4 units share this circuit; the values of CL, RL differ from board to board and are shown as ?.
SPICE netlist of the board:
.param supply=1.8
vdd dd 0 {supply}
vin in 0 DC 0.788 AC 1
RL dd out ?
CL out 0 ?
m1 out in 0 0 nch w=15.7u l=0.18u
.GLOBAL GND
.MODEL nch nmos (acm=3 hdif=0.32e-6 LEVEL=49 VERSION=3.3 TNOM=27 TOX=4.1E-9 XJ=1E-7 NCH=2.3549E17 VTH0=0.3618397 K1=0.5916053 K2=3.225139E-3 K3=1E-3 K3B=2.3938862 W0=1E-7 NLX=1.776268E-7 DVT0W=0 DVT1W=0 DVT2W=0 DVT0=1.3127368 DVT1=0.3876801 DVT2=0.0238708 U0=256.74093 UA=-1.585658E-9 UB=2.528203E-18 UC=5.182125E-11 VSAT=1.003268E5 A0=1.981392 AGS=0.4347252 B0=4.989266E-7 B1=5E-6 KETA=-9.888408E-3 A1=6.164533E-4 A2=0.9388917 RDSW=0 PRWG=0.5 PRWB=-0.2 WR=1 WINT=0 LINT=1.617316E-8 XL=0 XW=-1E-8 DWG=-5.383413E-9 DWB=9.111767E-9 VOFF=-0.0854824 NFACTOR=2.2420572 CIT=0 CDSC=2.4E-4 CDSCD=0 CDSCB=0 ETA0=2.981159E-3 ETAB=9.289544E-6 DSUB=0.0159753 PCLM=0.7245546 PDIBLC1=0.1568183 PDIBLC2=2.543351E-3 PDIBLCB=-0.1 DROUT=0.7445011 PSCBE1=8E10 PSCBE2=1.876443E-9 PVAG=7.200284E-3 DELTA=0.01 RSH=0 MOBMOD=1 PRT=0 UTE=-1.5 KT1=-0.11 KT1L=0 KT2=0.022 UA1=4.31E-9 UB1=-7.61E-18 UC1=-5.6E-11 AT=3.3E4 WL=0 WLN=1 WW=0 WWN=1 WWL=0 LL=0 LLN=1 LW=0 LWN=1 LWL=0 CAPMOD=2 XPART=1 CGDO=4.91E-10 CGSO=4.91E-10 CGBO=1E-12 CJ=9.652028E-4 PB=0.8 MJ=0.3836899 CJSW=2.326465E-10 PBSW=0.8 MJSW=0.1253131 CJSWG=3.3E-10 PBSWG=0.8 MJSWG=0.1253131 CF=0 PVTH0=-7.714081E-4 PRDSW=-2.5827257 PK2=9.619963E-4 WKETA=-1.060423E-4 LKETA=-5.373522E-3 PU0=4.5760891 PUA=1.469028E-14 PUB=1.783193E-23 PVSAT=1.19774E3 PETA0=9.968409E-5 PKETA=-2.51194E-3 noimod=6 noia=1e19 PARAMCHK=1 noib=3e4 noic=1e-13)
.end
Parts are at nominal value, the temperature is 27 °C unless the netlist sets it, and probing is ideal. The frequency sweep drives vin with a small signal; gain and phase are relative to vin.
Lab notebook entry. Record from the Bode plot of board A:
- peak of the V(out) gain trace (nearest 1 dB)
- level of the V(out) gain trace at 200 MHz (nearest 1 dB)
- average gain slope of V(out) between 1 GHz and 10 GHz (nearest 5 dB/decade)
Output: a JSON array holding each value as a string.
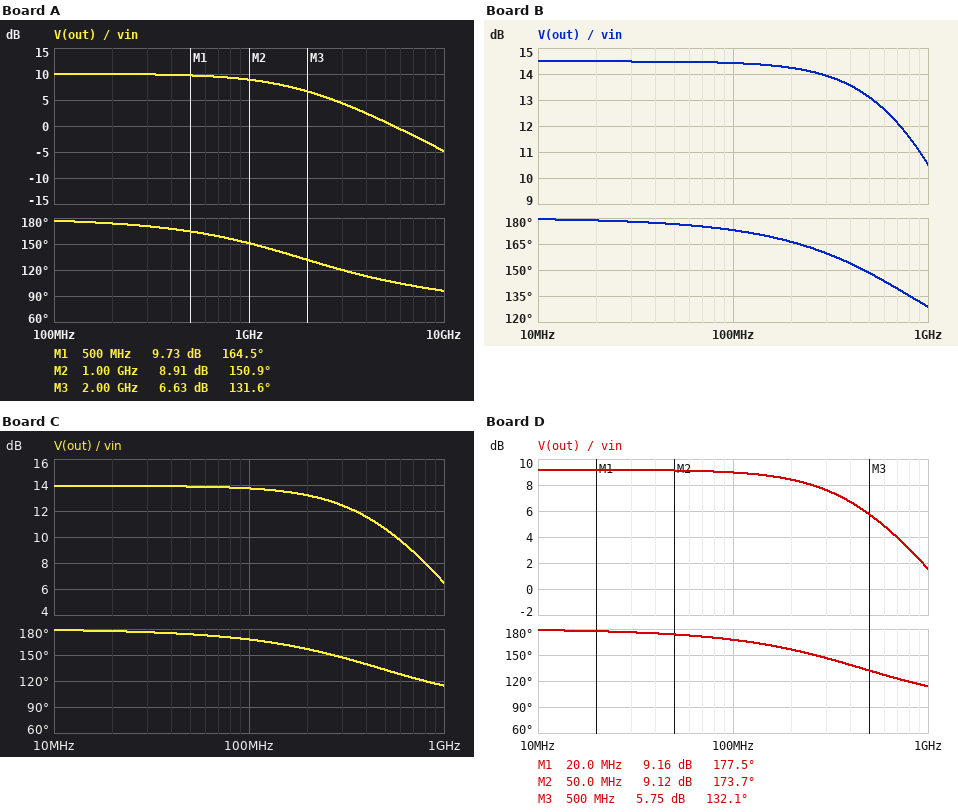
["10 dB", "10 dB", "-15 dB/decade"]
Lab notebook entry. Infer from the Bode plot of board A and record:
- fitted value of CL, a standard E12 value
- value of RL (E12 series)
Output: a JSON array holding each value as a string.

["150 fF", "560 Ω"]
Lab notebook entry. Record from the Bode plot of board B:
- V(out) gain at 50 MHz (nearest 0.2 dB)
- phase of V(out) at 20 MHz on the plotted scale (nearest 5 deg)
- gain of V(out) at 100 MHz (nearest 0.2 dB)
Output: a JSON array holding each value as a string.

["14.4 dB", "180 deg", "14.4 dB"]
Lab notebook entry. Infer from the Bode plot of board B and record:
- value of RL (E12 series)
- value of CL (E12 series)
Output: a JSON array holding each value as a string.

["1.5 kΩ", "180 fF"]
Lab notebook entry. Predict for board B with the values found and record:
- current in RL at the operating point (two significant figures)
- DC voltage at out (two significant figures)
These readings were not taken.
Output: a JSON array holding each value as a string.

["970 µA", "350 mV"]
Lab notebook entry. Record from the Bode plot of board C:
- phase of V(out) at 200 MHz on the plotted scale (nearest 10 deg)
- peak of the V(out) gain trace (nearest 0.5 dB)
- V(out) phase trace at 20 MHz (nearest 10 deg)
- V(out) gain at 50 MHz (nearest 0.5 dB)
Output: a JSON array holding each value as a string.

["160 deg", "14.0 dB", "180 deg", "14.0 dB"]
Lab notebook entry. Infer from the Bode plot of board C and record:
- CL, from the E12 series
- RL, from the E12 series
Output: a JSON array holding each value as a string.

["390 fF", "1 kΩ"]
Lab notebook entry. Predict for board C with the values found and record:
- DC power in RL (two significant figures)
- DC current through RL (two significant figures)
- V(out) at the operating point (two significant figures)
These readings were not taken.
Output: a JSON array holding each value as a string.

["1.1 mW", "1.1 mA", "730 mV"]
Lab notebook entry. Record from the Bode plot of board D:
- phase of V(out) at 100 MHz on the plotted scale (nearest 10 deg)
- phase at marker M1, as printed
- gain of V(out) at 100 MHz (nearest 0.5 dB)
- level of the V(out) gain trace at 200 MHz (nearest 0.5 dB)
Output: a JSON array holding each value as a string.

["170 deg", "177.5 deg", "9.0 dB", "8.5 dB"]
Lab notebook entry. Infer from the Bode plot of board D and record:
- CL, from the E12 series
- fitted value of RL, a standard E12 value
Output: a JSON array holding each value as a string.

["560 fF", "1.8 kΩ"]
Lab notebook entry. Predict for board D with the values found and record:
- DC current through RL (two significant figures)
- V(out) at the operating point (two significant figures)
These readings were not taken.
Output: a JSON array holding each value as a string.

["880 µA", "210 mV"]
